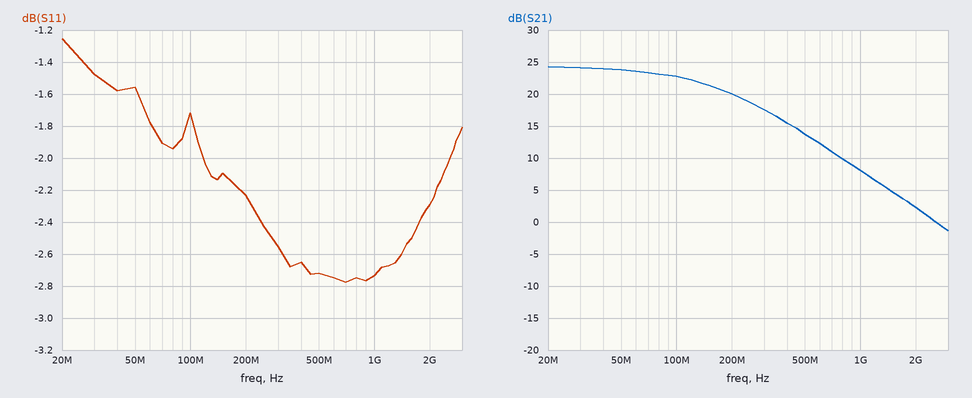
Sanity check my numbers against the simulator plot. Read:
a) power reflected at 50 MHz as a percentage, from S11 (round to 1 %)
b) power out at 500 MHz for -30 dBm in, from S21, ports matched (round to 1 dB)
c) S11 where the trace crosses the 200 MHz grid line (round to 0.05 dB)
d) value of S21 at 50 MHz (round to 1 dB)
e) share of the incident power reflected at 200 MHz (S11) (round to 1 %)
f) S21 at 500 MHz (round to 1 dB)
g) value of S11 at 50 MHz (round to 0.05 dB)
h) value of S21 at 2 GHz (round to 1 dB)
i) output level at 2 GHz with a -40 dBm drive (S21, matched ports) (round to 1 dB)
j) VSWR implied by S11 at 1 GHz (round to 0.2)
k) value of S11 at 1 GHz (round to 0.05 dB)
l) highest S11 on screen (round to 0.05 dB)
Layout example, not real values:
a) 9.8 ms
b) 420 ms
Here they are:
a) 70 %
b) -16 dBm
c) -2.25 dB
d) 24 dB
e) 60 %
f) 14 dB
g) -1.55 dB
h) 2 dB
i) -38 dBm
j) 6.4
k) -2.75 dB
l) -1.25 dB
